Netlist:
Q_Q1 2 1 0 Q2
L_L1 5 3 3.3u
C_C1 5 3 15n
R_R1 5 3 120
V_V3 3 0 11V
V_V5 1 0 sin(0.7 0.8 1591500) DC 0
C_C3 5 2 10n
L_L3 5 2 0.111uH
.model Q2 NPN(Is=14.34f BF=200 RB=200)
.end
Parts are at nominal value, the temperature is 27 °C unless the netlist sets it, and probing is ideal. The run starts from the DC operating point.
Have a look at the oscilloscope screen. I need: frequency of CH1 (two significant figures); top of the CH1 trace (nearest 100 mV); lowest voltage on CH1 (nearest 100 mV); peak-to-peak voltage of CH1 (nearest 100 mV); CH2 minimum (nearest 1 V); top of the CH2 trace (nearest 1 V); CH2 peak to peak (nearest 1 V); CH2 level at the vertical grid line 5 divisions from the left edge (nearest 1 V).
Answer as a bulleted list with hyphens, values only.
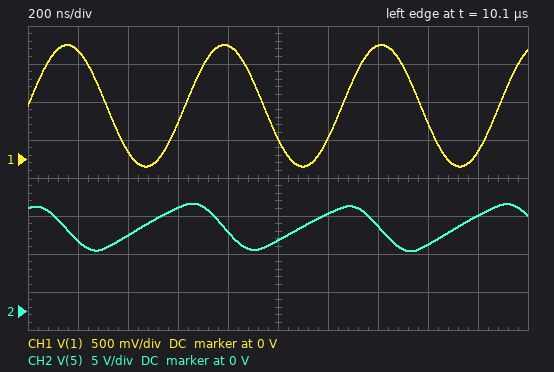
- 1.6 MHz
- 1.5 V
- -100 mV
- 1.6 V
- 8 V
- 14 V
- 6 V
- 9 V
